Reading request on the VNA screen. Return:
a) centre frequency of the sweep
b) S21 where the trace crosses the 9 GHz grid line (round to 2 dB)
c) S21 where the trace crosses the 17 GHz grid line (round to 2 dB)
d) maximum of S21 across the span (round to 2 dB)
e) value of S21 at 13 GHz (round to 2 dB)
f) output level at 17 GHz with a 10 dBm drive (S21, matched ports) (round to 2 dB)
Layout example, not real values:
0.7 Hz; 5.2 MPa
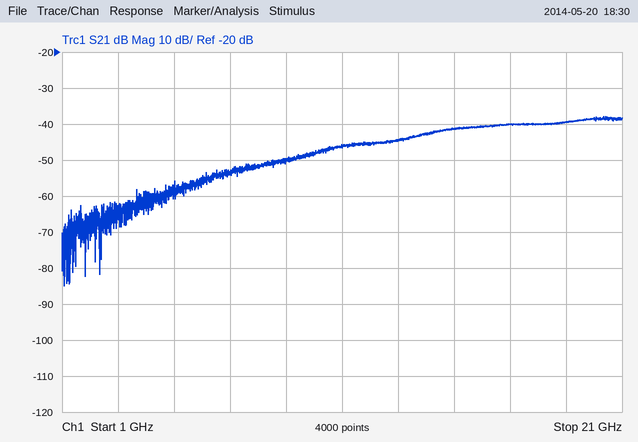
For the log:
11 GHz; -50 dB; -40 dB; -38 dB; -44 dB; -30 dBm
